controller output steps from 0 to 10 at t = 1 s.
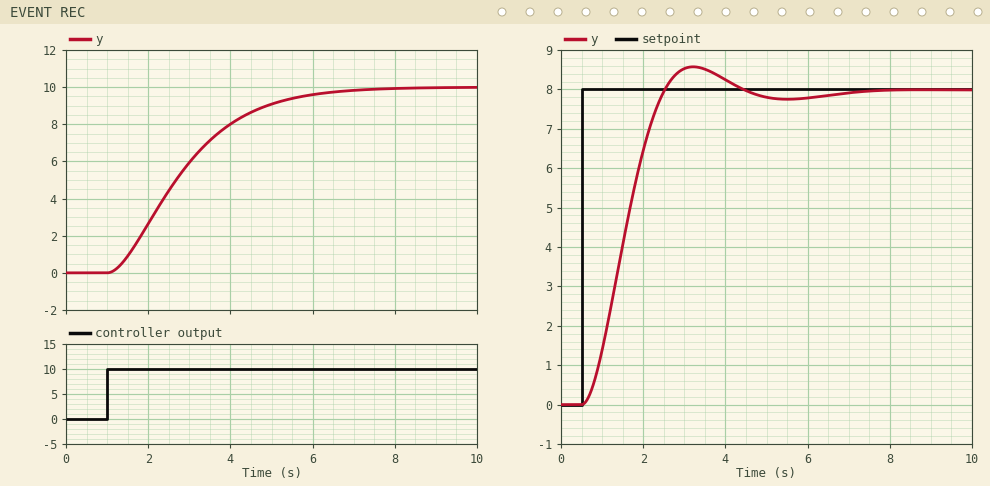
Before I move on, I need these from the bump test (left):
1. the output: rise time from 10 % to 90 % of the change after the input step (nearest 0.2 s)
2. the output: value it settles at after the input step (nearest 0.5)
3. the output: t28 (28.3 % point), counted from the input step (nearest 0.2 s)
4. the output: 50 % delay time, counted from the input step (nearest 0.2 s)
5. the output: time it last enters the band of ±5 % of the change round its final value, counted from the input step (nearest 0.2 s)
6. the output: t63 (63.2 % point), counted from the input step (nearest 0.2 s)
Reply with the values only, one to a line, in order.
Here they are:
3.4 s
10.0
1.0 s
1.6 s
4.8 s
2.2 s
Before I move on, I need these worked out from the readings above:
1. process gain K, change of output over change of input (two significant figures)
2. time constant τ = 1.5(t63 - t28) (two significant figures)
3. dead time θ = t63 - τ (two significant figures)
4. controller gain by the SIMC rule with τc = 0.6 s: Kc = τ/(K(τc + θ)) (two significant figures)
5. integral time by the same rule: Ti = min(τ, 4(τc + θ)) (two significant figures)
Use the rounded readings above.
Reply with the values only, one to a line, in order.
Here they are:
1.0
1.8 s
0.40 s
1.8
1.8 s
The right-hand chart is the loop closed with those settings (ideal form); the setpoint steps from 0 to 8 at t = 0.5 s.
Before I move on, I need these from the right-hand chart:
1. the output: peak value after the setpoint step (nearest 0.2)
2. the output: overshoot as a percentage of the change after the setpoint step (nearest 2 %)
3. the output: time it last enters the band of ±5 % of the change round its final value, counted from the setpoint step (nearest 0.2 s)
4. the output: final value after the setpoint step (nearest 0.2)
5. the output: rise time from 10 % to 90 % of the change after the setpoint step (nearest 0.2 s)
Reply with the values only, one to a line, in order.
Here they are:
8.6
8 %
3.2 s
8.0
1.4 s
